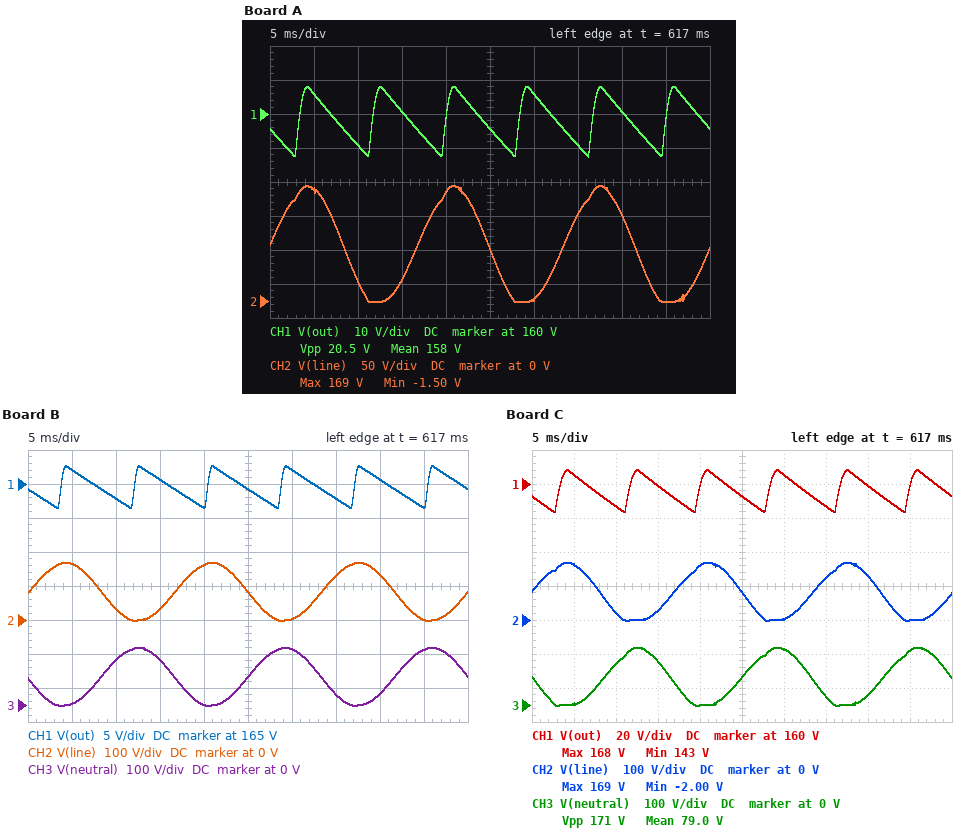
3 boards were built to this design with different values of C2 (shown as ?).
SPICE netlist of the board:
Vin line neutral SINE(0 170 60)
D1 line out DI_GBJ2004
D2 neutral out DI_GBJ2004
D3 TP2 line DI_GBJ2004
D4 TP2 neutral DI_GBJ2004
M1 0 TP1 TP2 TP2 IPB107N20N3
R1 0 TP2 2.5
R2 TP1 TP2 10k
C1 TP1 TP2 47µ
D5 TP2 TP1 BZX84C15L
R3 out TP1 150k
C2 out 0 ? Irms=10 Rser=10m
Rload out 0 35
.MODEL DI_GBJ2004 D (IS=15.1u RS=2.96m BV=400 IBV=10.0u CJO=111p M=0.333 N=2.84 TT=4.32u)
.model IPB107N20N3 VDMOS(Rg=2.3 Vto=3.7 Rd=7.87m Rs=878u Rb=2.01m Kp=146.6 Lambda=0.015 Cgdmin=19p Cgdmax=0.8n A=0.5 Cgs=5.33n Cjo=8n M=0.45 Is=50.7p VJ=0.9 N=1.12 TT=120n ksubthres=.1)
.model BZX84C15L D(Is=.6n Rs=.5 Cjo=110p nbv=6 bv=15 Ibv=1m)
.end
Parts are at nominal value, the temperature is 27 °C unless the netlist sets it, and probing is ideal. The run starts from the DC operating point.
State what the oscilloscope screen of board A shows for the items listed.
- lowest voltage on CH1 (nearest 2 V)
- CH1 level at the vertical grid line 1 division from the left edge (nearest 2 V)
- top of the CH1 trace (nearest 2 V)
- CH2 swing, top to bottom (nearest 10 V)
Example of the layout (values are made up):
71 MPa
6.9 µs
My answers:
148 V
166 V
168 V
170 V
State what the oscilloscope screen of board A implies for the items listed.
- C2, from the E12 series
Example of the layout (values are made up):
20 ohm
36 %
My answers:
1.5 mF
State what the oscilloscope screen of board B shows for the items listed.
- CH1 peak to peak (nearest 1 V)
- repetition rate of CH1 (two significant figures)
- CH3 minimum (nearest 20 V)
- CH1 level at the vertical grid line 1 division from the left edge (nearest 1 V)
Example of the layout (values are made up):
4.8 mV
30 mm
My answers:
6 V
120 Hz
0 V
167 V
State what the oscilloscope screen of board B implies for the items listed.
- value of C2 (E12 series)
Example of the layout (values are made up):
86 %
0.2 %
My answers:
5.6 mF
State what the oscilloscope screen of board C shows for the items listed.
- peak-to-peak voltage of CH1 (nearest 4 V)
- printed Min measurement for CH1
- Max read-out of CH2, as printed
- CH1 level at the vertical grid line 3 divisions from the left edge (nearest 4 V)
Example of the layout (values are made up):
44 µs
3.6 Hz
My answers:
24 V
143 V
169 V
160 V
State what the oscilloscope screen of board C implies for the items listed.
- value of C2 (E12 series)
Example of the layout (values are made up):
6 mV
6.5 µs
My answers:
1.2 mF
